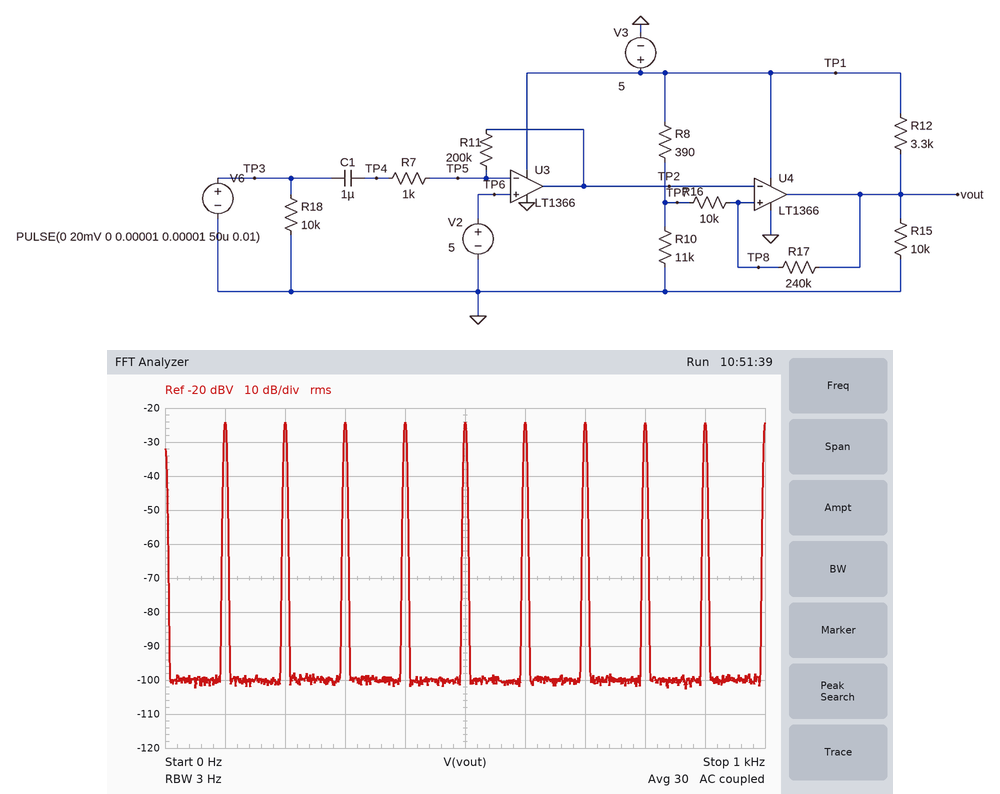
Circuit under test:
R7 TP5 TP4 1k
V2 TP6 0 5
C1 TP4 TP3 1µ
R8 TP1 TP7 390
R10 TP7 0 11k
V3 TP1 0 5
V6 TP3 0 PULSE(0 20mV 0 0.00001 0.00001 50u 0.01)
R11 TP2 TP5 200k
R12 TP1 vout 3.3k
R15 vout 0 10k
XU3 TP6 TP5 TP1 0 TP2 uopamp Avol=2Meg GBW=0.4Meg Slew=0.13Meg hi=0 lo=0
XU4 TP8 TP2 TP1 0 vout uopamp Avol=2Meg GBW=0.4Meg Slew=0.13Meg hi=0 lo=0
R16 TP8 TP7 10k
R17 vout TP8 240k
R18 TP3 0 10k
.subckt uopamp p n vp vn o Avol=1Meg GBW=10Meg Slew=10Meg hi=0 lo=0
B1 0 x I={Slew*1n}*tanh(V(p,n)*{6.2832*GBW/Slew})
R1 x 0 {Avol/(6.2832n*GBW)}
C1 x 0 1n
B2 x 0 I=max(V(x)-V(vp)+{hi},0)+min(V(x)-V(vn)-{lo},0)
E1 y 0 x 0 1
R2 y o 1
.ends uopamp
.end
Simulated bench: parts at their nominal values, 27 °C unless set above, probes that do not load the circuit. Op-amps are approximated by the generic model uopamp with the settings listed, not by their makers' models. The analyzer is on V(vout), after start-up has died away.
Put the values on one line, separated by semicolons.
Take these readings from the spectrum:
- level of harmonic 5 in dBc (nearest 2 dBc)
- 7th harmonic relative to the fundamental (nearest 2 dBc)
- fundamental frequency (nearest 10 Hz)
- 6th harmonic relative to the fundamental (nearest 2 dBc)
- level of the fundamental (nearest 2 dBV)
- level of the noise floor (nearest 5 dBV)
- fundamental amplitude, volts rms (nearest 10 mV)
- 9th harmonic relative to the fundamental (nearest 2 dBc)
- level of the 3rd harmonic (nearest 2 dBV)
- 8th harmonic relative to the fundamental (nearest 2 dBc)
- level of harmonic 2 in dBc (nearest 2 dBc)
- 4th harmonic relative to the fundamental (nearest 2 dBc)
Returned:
0 dBc; 0 dBc; 100 Hz; 0 dBc; -24 dBV; -100 dBV; 60 mV; 0 dBc; -24 dBV; 0 dBc; 0 dBc; 0 dBc
